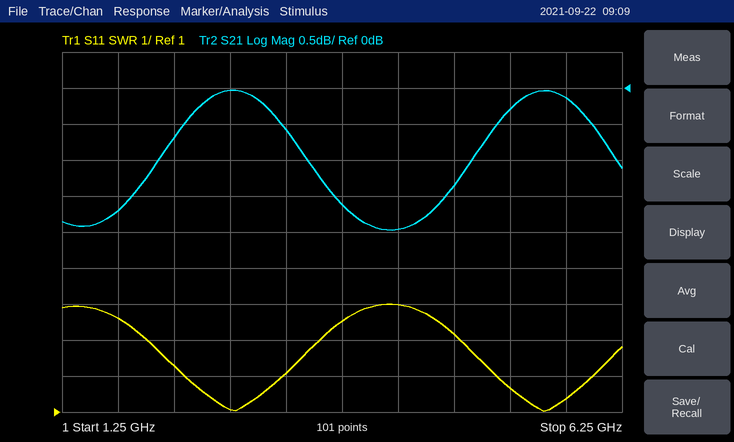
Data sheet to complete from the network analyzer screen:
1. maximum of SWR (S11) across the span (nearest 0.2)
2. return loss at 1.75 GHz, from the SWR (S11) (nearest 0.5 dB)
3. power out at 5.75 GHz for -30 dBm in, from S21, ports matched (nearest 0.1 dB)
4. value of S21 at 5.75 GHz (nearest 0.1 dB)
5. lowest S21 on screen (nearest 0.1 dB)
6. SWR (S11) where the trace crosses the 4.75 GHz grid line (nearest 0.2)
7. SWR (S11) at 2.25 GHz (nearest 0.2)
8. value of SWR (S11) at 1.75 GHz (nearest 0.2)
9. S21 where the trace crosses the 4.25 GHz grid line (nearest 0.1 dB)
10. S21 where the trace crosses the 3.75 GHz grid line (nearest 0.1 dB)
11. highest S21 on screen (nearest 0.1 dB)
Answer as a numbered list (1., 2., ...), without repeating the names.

1. 4.0
2. 5.0 dB
3. -30.1 dBm
4. -0.1 dB
5. -2.0 dB
6. 3.2
7. 2.2
8. 3.6
9. -2.0 dB
10. -1.6 dB
11. 0.0 dB
